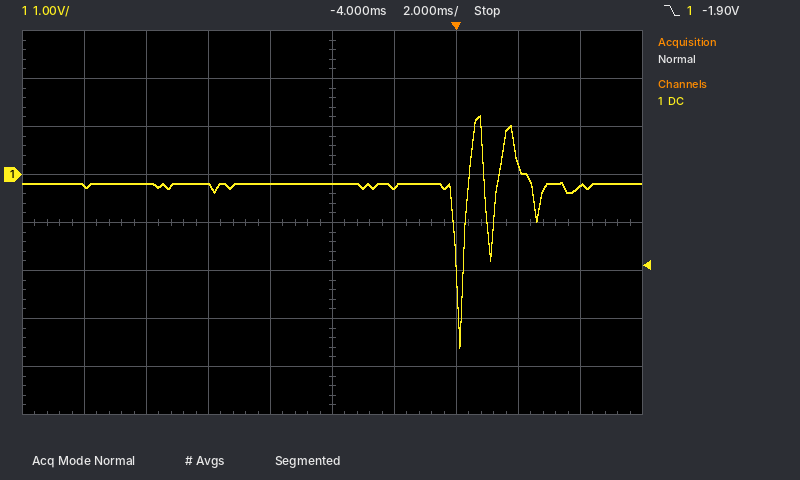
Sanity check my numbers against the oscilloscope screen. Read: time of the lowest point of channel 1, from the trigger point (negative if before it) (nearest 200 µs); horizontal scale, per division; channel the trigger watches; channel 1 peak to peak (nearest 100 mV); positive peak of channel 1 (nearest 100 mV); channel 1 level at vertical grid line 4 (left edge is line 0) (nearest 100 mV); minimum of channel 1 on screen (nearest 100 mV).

+200 µs
2 ms
channel 1
4.8 V
1.2 V
-200 mV
-3.6 V
